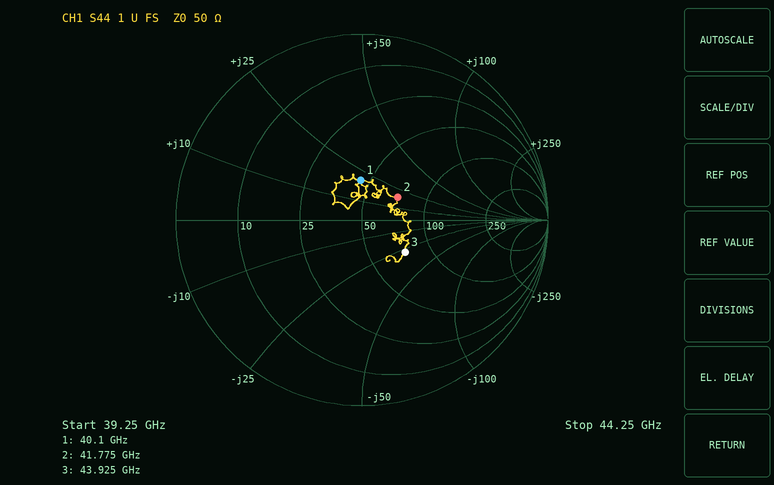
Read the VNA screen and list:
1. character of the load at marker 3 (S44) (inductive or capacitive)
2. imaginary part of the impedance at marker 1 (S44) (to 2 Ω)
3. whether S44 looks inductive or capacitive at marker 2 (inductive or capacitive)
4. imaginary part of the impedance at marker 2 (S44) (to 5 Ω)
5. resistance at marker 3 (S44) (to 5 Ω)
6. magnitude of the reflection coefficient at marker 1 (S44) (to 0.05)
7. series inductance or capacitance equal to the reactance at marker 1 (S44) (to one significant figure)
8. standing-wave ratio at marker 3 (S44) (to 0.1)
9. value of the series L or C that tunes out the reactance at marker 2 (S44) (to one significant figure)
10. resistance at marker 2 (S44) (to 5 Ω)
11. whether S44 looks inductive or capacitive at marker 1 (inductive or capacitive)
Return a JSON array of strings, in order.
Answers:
["capacitive", "+20 Ω", "inductive", "+20 Ω", "75 Ω", "0.20", "80 pH", "1.8", "200 fF", "70 Ω", "inductive"]
